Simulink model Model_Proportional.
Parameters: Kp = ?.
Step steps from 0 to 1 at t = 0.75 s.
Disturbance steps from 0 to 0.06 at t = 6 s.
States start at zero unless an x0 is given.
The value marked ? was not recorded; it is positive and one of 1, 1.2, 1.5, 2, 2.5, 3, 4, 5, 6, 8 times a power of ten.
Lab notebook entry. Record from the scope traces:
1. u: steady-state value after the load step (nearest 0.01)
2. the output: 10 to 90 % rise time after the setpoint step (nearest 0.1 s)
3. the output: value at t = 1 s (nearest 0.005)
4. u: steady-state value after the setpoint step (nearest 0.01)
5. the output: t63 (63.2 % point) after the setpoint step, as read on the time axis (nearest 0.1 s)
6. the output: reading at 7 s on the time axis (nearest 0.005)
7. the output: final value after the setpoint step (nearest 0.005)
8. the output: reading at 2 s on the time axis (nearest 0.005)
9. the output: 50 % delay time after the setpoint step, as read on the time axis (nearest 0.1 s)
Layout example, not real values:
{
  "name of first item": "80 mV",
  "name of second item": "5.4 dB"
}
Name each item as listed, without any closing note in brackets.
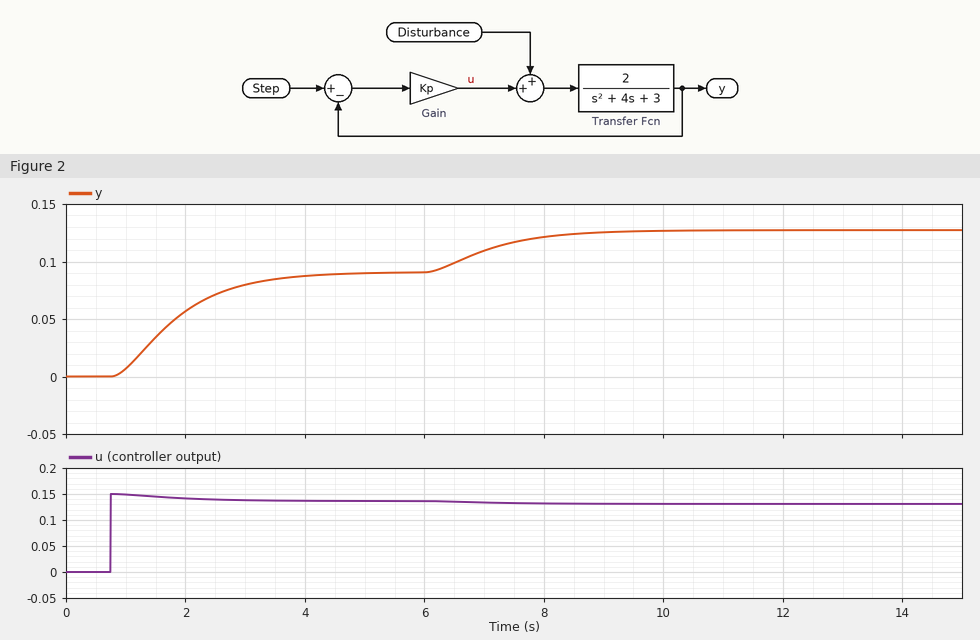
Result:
{
  "u: steady-state value after the load step": "0.13",
  "the output: 10 to 90 % rise time after the setpoint step": "2.1 s",
  "the output: value at t = 1 s": "0.005",
  "u: steady-state value after the setpoint step": "0.14",
  "the output: t63 (63.2 % point) after the setpoint step, as read on the time axis": "2.0 s",
  "the output: reading at 7 s on the time axis": "0.110",
  "the output: final value after the setpoint step": "0.090",
  "the output: reading at 2 s on the time axis": "0.055",
  "the output: 50 % delay time after the setpoint step, as read on the time axis": "1.7 s"
}
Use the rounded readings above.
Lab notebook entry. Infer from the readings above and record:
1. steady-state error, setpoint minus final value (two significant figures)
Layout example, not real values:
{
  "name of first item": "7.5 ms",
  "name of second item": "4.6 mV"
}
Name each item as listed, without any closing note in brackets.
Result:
{
  "steady-state error, setpoint minus final value": "0.91"
}
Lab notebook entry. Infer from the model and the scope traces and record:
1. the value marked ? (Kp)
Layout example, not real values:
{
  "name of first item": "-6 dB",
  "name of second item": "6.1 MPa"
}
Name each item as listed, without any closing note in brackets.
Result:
{
  "the value marked ?": "0.15"
}
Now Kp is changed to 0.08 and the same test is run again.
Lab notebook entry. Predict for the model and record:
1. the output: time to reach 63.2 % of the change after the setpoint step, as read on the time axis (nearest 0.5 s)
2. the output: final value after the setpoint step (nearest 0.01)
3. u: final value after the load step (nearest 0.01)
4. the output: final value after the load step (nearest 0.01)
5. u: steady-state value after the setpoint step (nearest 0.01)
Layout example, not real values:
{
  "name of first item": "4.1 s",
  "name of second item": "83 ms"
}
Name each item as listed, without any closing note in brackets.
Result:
{
  "the output: time to reach 63.2 % of the change after the setpoint step, as read on the time axis": "2.0 s",
  "the output: final value after the setpoint step": "0.05",
  "u: final value after the load step": "0.07",
  "the output: final value after the load step": "0.09",
  "u: steady-state value after the setpoint step": "0.08"
}
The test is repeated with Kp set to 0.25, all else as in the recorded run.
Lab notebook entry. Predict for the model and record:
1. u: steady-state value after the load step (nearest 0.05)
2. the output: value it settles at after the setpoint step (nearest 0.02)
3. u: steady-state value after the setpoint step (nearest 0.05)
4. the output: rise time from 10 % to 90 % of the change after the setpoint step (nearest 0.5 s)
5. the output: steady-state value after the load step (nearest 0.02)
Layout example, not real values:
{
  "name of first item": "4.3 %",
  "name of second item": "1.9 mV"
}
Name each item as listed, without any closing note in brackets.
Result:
{
  "u: steady-state value after the load step": "0.20",
  "the output: value it settles at after the setpoint step": "0.14",
  "u: steady-state value after the setpoint step": "0.20",
  "the output: rise time from 10 % to 90 % of the change after the setpoint step": "2.0 s",
  "the output: steady-state value after the load step": "0.18"
}
